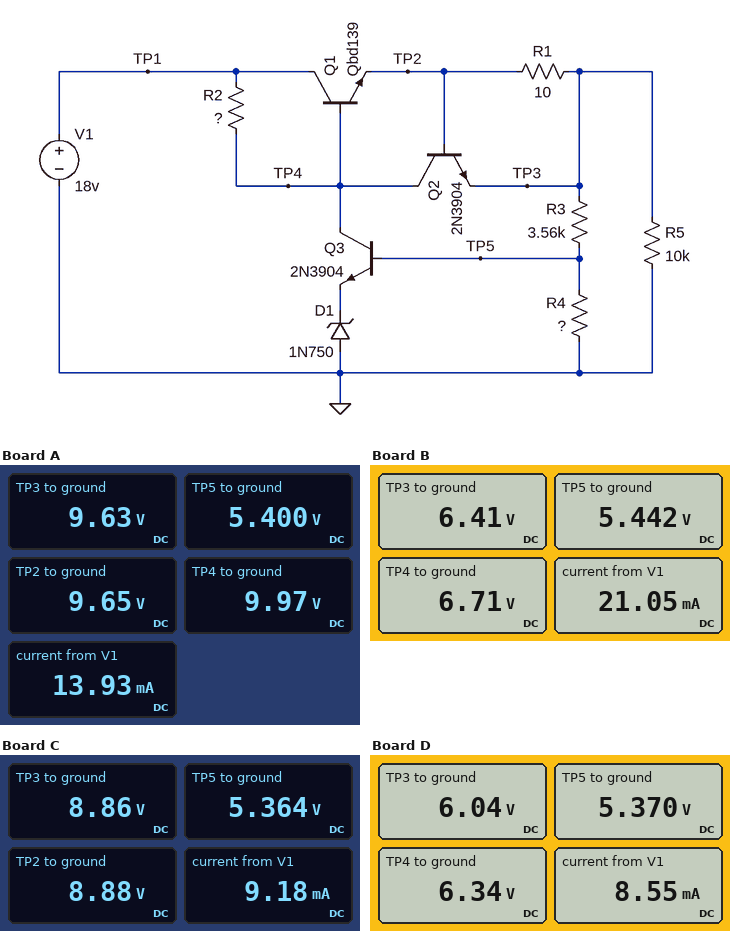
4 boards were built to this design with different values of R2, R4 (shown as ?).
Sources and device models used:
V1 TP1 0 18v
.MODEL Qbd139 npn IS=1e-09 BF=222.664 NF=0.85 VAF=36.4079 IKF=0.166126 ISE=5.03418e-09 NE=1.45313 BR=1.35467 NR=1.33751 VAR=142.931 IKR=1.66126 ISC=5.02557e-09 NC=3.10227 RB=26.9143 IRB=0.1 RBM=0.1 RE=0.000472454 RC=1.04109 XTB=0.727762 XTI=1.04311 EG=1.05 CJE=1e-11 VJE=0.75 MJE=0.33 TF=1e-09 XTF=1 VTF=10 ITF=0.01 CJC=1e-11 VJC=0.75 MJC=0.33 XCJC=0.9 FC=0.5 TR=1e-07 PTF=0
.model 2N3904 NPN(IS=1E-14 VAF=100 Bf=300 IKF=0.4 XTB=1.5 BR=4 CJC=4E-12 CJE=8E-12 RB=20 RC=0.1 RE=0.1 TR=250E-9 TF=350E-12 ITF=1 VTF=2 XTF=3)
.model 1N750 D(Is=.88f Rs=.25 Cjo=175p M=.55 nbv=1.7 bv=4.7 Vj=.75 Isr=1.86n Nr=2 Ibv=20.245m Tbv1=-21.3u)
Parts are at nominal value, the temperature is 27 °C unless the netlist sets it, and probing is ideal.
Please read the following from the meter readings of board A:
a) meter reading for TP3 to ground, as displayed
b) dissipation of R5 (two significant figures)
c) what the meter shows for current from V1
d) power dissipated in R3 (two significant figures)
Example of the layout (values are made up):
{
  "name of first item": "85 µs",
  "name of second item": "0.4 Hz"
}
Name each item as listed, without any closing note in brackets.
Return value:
{
  "meter reading for TP3 to ground, as displayed": "9.63 V",
  "dissipation of R5": "9.3 mW",
  "what the meter shows for current from V1": "13.93 mA",
  "power dissipated in R3": "5.0 mW"
}
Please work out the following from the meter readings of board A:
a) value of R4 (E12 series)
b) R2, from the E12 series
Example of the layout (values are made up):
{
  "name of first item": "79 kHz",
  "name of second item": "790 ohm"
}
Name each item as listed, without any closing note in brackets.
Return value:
{
  "value of R4": "4.7 kΩ",
  "R2, from the E12 series": "680 Ω"
}
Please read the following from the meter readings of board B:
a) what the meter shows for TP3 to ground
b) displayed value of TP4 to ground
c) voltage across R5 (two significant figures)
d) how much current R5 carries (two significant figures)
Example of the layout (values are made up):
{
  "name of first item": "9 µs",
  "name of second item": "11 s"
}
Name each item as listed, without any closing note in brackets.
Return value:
{
  "what the meter shows for TP3 to ground": "6.41 V",
  "displayed value of TP4 to ground": "6.71 V",
  "voltage across R5": "6.4 V",
  "how much current R5 carries": "640 µA"
}
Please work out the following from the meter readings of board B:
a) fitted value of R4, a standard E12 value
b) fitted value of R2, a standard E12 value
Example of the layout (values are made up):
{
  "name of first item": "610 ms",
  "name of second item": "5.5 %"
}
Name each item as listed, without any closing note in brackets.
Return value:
{
  "fitted value of R4, a standard E12 value": "27 kΩ",
  "fitted value of R2, a standard E12 value": "560 Ω"
}
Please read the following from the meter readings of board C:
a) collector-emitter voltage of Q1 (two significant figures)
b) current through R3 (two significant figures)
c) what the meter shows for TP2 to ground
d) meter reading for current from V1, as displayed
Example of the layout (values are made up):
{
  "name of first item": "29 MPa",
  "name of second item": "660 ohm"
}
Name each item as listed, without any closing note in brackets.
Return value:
{
  "collector-emitter voltage of Q1": "9.1 V",
  "current through R3": "980 µA",
  "what the meter shows for TP2 to ground": "8.88 V",
  "meter reading for current from V1, as displayed": "9.18 mA"
}
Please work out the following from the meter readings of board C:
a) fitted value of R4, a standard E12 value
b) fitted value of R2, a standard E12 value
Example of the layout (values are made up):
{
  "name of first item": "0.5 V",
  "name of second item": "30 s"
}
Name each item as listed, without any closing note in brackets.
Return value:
{
  "fitted value of R4, a standard E12 value": "5.6 kΩ",
  "fitted value of R2, a standard E12 value": "1.2 kΩ"
}
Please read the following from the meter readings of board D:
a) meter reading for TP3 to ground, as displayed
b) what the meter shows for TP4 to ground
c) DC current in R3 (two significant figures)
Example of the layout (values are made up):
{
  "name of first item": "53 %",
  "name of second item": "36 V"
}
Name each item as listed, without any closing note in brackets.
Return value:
{
  "meter reading for TP3 to ground, as displayed": "6.04 V",
  "what the meter shows for TP4 to ground": "6.34 V",
  "DC current in R3": "190 µA"
}
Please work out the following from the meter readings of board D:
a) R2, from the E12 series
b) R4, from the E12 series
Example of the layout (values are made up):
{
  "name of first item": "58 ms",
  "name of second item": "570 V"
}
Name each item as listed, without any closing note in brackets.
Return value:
{
  "R2, from the E12 series": "1.5 kΩ",
  "R4, from the E12 series": "33 kΩ"
}
